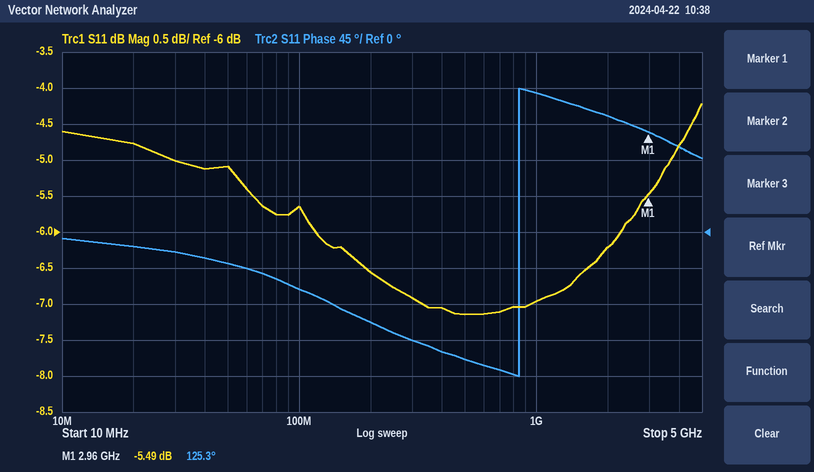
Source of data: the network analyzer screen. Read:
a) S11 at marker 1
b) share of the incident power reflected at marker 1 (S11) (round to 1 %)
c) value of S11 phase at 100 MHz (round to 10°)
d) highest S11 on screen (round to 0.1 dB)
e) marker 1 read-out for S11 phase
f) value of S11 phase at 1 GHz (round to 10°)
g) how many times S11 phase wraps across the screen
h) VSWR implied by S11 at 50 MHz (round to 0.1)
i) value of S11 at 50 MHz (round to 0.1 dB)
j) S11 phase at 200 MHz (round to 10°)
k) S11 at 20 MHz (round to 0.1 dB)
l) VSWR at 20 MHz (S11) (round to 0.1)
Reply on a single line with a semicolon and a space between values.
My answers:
-5.49 dB; 28 %; -70°; -4.2 dB; 125.3°; 170°; 1; 3.5; -5.1 dB; -110°; -4.8 dB; 3.7
